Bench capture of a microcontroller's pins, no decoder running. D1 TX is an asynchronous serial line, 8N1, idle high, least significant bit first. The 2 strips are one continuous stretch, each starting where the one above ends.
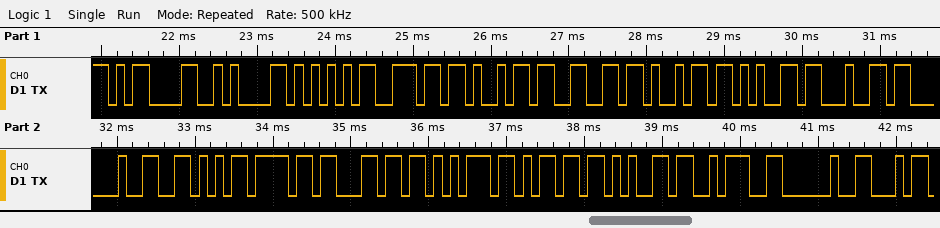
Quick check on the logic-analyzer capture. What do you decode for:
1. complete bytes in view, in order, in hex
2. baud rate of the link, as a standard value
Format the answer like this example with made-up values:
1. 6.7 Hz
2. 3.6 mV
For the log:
1. 0D 0A 55 6E 69 66 69 65 64 20 56 6F 6C 75 6D 65 3A 20
2. 9600 baud
